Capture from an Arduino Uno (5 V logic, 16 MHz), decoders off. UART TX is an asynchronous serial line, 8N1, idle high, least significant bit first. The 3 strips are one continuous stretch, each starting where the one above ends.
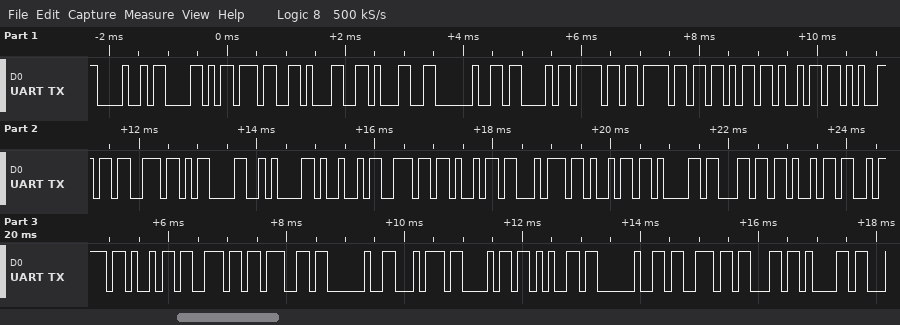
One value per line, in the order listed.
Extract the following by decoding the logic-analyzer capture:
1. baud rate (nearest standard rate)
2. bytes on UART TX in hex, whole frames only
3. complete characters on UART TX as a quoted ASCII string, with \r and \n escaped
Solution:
9600 baud
48 58 37 31 31 20 43 6F 6F 6B 69 65 73 0D 0A 49 6E 69 74 69 61 6C 69 7A 69 6E 67 20 74 68 65 20 73 63 61
"HX711 Cookies\r\nInitializing the sca"
